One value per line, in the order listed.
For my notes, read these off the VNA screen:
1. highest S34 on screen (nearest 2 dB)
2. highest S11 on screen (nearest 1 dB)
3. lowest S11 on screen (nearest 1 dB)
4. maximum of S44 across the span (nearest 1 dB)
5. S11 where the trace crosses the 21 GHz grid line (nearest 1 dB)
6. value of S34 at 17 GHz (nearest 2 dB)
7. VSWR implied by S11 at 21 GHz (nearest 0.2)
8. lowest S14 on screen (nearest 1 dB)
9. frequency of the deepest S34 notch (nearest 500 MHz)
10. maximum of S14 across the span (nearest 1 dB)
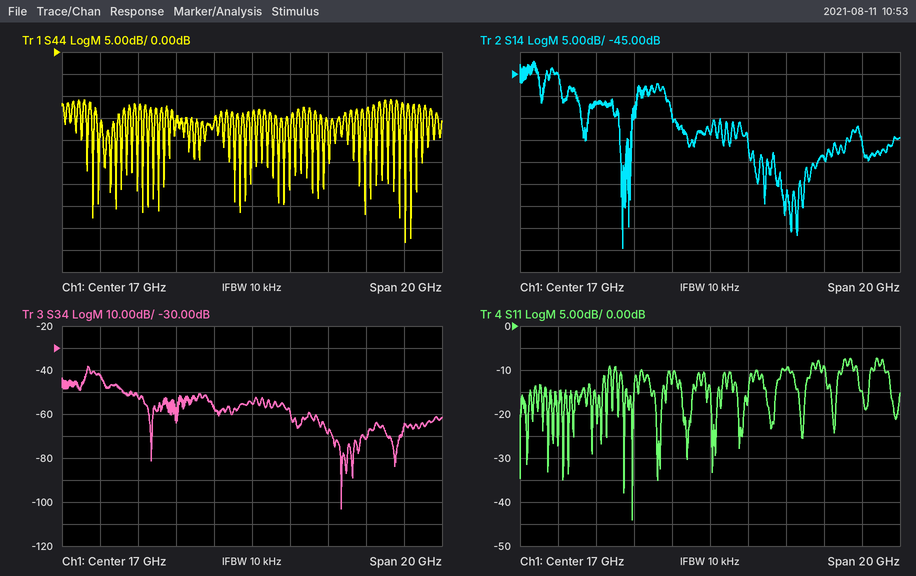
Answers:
-38 dB
-7 dB
-44 dB
-11 dB
-10 dB
-56 dB
2.0
-85 dB
21.5 GHz
-42 dB
